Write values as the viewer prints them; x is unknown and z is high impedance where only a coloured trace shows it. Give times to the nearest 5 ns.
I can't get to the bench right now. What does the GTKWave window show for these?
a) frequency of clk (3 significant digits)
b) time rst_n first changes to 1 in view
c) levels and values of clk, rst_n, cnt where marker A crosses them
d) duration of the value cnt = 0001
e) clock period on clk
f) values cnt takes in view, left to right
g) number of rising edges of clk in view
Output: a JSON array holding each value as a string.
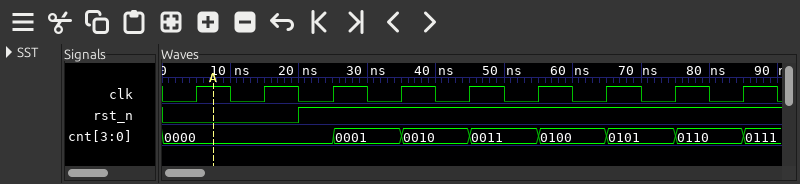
["100 MHz", "20 ns", "clk=1, rst_n=0, cnt=0000", "10 ns", "10 ns", "0000, 0001, 0010, 0011, 0100, 0101, 0110, 0111", "9"]
